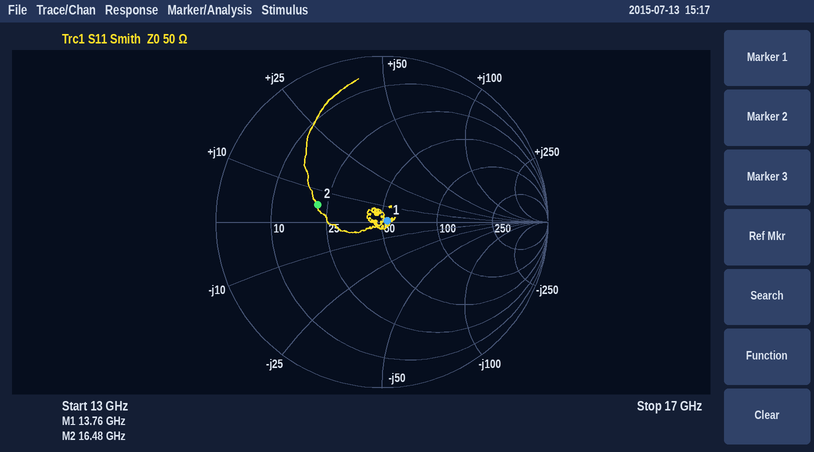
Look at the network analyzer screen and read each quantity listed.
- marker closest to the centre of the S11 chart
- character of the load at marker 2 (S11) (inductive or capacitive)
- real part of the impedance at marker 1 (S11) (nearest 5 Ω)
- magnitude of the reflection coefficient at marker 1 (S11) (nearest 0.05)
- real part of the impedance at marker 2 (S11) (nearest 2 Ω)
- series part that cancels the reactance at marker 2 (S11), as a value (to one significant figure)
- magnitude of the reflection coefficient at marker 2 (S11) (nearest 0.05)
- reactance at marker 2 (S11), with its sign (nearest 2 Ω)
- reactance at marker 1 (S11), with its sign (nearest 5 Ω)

marker 1
inductive
55 Ω
0.05
22 Ω
2 pF
0.40
+6 Ω
0 Ω
